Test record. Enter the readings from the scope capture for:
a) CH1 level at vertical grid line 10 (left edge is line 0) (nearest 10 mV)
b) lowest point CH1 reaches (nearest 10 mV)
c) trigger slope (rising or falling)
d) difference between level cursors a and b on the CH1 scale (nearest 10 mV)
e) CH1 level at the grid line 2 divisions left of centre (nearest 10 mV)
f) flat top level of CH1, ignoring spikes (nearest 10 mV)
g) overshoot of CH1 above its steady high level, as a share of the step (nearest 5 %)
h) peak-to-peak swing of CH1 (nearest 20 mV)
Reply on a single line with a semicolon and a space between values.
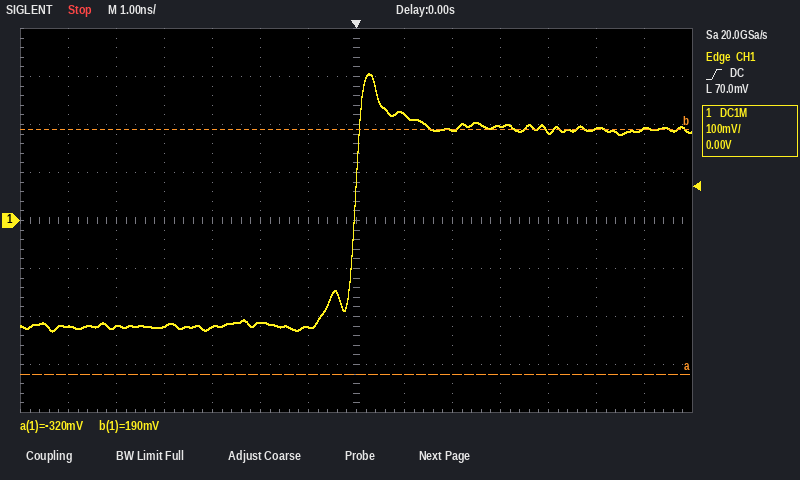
200 mV; -230 mV; rising; 510 mV; -210 mV; 190 mV; 30 %; 540 mV
